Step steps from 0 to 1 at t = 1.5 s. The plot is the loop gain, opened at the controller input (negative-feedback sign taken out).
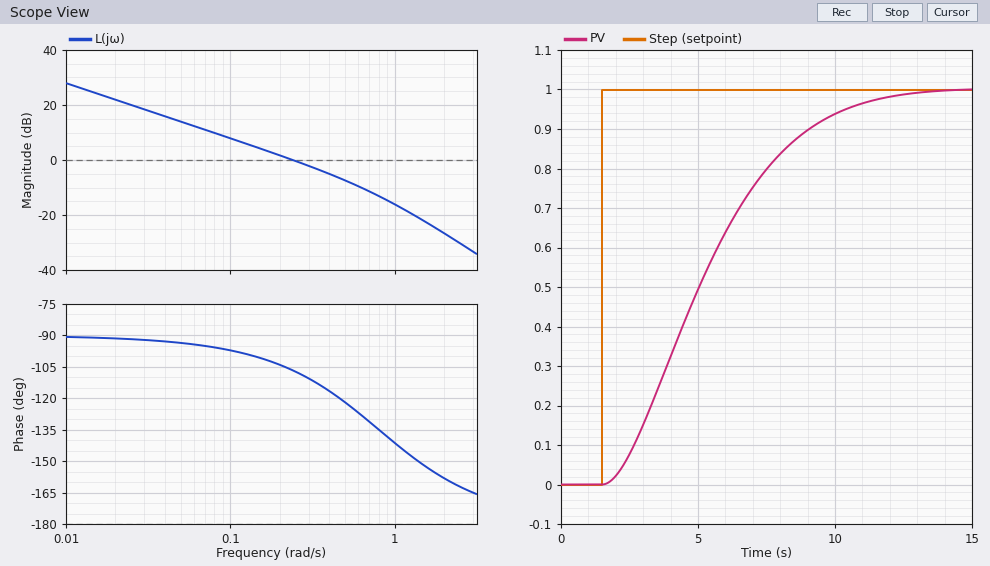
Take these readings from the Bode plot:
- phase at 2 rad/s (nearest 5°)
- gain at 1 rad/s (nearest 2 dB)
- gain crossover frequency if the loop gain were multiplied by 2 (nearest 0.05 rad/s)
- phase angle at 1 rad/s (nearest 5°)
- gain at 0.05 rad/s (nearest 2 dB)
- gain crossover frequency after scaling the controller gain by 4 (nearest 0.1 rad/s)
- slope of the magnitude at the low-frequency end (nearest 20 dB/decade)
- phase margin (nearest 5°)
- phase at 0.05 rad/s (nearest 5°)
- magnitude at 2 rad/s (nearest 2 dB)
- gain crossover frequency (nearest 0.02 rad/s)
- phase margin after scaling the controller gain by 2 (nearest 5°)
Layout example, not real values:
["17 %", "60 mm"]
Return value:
["-160°", "-16 dB", "0.45 rad/s", "-140°", "14 dB", "0.7 rad/s", "-20 dB/decade", "75°", "-95°", "-26 dB", "0.24 rad/s", "60°"]
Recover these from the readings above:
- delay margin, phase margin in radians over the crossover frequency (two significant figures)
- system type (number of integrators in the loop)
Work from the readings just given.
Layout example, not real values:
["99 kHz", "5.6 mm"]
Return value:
["5.5 s", "1"]
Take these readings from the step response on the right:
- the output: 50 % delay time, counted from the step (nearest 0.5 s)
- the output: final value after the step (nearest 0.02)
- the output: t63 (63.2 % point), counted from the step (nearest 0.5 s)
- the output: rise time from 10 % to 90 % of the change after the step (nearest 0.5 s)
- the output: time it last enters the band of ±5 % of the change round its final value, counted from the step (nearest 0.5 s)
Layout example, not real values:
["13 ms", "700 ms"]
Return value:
["3.5 s", "1.00", "4.5 s", "6.5 s", "9.0 s"]
